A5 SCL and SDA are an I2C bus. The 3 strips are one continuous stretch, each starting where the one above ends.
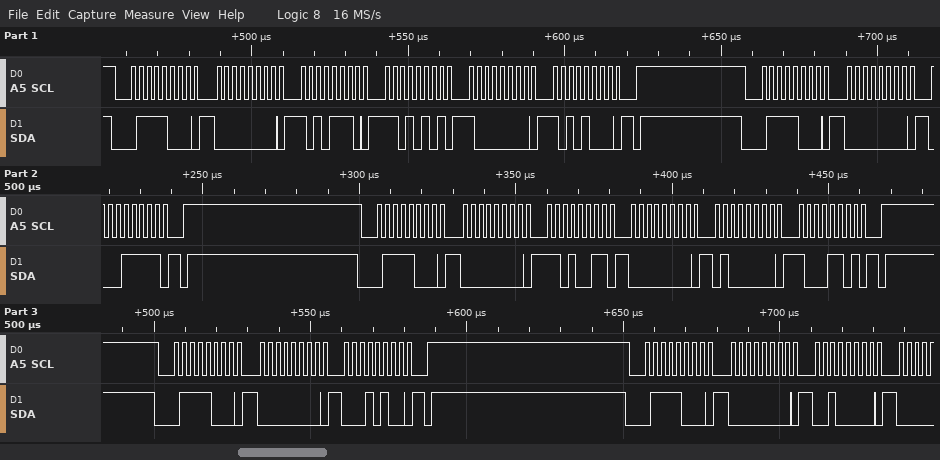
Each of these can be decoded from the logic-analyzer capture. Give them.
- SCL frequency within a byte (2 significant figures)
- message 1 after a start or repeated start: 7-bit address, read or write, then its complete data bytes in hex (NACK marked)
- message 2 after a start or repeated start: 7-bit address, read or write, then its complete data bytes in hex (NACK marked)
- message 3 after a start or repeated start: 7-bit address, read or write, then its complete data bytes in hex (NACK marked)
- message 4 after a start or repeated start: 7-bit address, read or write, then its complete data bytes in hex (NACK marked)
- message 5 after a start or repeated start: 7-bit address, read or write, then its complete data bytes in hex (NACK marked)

400 kHz
0x3C write: 00 AE D5 80 A8
0x3C write: 00 1F
0x3C write: 00 D3 00 40 8D
0x3C write: 00 14
0x3C write: 00 20
